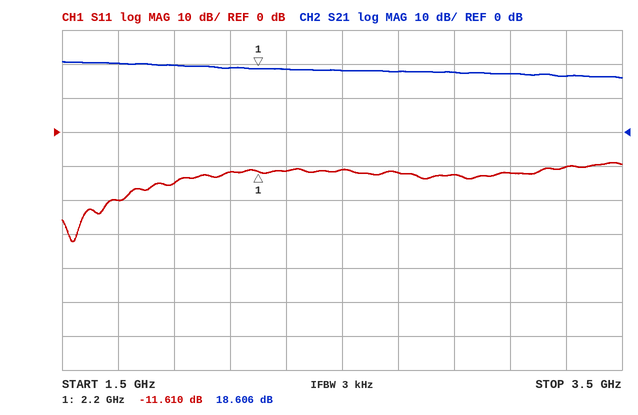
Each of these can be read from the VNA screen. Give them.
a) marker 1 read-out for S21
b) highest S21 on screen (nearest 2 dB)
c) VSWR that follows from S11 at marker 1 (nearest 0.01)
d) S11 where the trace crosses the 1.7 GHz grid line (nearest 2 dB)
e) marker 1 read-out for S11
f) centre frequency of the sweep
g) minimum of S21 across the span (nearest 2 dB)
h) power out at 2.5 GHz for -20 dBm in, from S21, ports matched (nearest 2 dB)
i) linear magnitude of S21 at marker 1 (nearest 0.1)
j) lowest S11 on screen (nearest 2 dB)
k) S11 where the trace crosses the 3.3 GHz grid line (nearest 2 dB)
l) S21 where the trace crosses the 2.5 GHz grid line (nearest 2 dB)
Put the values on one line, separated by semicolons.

18.606 dB; 20 dB; 1.71; -20 dB; -11.610 dB; 2.5 GHz; 16 dB; -2 dBm; 8.5; -32 dB; -10 dB; 18 dB
